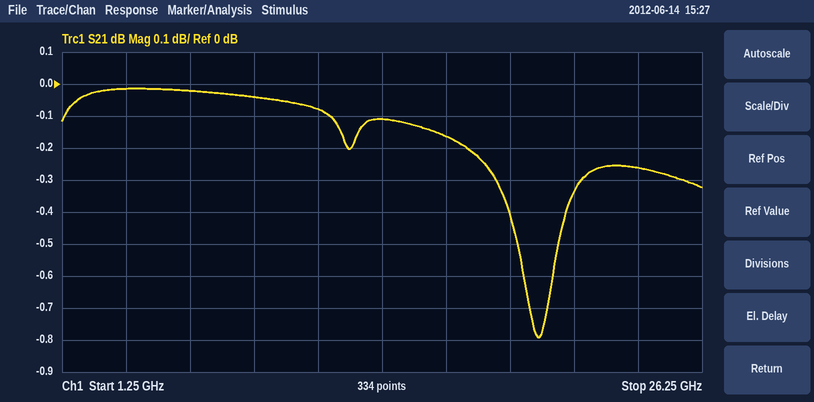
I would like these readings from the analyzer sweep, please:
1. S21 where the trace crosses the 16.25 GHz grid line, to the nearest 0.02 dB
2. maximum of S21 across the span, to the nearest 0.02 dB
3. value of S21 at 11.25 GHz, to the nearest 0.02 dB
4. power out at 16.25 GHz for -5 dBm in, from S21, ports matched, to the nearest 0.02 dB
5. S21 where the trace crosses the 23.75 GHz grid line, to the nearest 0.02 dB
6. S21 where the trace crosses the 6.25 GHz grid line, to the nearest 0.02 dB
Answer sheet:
-0.16 dB
-0.02 dB
-0.08 dB
-5.16 dBm
-0.26 dB
-0.02 dB
